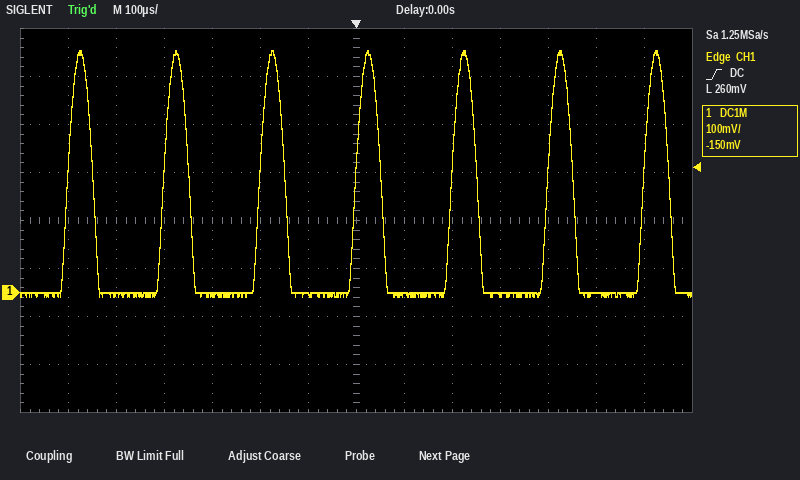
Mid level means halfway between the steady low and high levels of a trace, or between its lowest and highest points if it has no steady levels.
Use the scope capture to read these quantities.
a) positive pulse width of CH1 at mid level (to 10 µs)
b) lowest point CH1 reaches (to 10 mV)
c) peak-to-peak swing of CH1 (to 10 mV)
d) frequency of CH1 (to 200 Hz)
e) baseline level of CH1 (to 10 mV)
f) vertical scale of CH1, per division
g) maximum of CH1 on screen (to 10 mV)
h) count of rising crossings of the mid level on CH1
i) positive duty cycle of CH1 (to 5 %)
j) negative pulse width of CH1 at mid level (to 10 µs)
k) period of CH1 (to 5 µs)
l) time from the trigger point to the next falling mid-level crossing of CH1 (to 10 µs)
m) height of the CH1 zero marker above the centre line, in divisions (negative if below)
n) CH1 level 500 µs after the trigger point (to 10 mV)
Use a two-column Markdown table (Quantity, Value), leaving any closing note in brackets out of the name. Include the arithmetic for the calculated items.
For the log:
| Quantity | Value |
|---|---|
| positive pulse width of CH1 at mid level | 50 µs |
| lowest point CH1 reaches | -10 mV |
| peak-to-peak swing of CH1 | 500 mV − (-10 mV) = 510 mV |
| frequency of CH1 | 1 / 200 µs ≈ 5.0 kHz |
| baseline level of CH1 | 0 mV |
| vertical scale of CH1, per division | 100 mV |
| maximum of CH1 on screen | 500 mV |
| count of rising crossings of the mid level on CH1 | 7 |
| positive duty cycle of CH1 | 50 µs / 200 µs ≈ 25 % |
| negative pulse width of CH1 at mid level | 150 µs |
| period of CH1 | 200 µs |
| time from the trigger point to the next falling mid-level crossing of CH1 | 50 µs |
| height of the CH1 zero marker above the centre line, in divisions | -1.5 div |
| CH1 level 500 µs after the trigger point | 0 mV |
